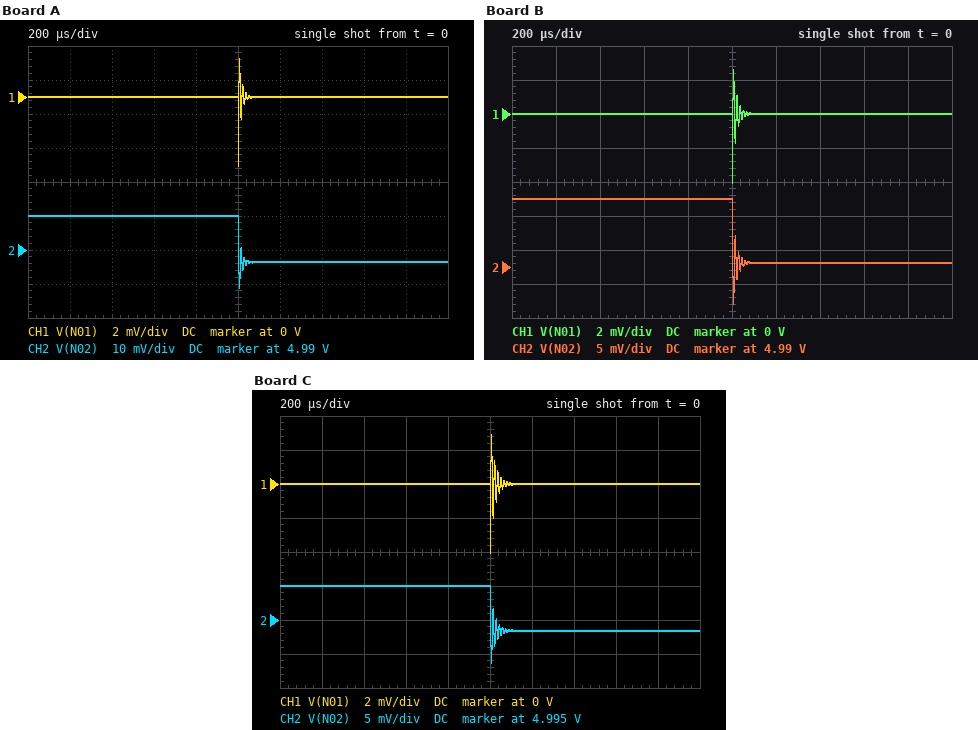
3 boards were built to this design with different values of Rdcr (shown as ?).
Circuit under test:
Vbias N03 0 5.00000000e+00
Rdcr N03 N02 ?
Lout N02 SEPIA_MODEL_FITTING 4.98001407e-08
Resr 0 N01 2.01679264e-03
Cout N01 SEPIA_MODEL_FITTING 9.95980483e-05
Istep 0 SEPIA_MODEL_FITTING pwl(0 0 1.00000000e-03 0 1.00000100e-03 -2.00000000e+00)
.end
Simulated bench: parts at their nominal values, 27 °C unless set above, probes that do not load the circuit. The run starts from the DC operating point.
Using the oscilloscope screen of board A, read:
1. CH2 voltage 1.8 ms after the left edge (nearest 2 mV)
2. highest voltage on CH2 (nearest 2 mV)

4.986 V
5.000 V
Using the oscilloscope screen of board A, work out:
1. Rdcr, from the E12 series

6.8 mΩ
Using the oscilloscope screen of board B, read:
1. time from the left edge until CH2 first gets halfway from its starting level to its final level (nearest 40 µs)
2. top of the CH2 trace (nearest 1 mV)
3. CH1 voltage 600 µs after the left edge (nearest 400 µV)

1.00 ms
5.000 V
0 V
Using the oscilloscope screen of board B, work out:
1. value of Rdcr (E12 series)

4.7 mΩ
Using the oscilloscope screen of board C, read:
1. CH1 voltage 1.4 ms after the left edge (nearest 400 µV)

0 V
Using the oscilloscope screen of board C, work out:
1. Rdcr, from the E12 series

3.3 mΩ
